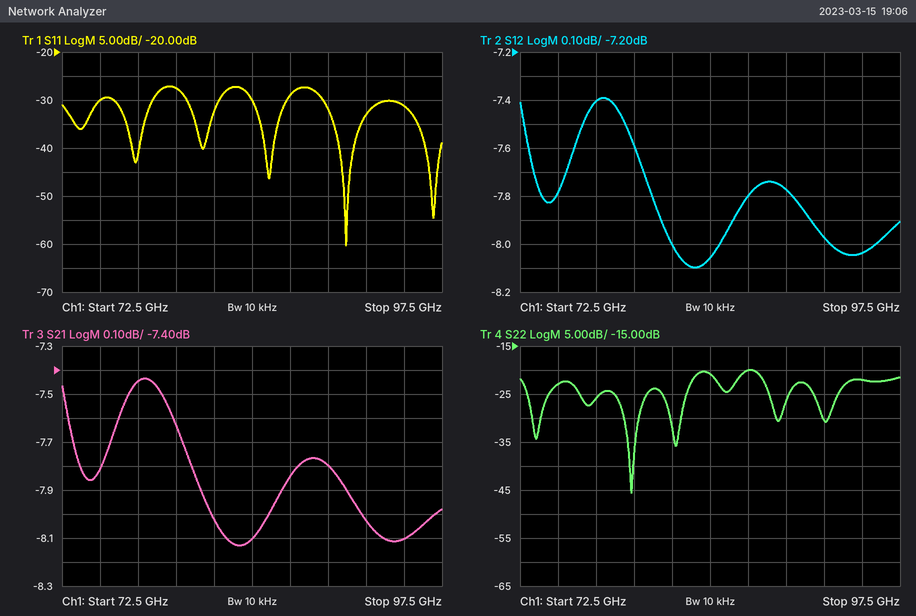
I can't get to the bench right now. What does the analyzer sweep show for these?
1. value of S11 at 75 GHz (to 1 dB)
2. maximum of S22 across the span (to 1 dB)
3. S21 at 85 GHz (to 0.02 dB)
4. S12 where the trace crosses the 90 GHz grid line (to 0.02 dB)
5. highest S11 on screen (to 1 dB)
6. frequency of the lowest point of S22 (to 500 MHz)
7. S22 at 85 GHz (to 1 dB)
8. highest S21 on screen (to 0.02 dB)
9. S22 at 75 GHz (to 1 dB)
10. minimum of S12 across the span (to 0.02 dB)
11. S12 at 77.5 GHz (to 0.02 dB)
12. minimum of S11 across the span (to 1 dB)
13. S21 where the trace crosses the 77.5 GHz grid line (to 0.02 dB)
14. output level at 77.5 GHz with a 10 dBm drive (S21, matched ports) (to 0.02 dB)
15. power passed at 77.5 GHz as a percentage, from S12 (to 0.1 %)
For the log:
-30 dB
-20 dB
-8.10 dB
-7.78 dB
-27 dB
80.0 GHz
-21 dB
-7.44 dB
-23 dB
-8.10 dB
-7.40 dB
-60 dB
-7.44 dB
2.56 dBm
18.2 %
